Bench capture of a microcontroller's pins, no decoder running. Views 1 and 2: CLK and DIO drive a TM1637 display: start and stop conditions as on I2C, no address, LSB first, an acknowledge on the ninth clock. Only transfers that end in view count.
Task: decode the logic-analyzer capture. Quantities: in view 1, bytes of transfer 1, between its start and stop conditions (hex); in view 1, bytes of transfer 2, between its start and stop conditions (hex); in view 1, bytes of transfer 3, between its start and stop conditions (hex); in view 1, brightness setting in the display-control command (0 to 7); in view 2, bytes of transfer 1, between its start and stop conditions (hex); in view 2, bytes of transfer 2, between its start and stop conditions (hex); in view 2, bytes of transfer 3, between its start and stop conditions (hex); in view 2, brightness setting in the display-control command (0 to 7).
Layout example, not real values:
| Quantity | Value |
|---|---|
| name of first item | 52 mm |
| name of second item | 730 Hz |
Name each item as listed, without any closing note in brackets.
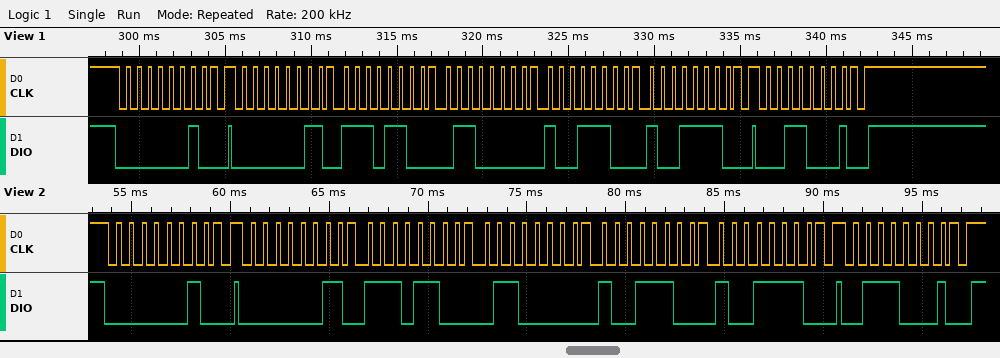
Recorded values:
| Quantity | Value |
|---|---|
| in view 1, bytes of transfer 1, between its start and stop conditions | 40 |
| in view 1, bytes of transfer 2, between its start and stop conditions | C0 37 06 39 79 |
| in view 1, bytes of transfer 3, between its start and stop conditions | 8C |
| in view 1, brightness setting in the display-control command | 4 |
| in view 2, bytes of transfer 1, between its start and stop conditions | 40 |
| in view 2, bytes of transfer 2, between its start and stop conditions | C0 37 06 39 79 |
| in view 2, bytes of transfer 3, between its start and stop conditions | 8E |
| in view 2, brightness setting in the display-control command | 6 |
